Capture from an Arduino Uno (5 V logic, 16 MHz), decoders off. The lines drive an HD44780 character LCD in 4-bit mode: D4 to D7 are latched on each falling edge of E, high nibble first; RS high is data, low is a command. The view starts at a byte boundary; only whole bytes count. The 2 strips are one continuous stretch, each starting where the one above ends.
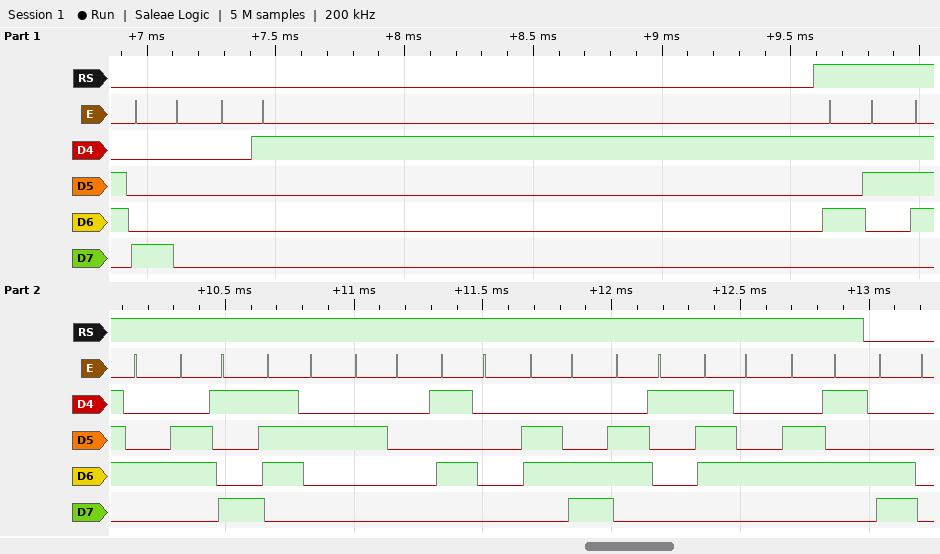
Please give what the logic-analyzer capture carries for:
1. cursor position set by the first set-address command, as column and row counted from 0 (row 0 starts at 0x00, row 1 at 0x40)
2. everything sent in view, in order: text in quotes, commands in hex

column 0, row 0
0x80 0x01 "Stir Plate" 0xC0
